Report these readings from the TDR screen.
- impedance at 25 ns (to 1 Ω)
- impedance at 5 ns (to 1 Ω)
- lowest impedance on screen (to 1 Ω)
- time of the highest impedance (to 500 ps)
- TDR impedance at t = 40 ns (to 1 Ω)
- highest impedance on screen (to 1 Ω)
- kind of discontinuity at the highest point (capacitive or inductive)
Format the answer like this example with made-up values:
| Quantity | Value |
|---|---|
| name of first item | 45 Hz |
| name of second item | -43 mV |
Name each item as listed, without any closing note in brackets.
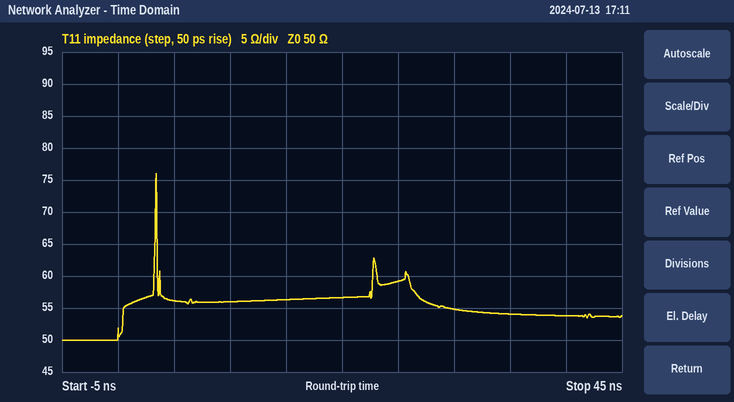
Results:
| Quantity | Value |
|---|---|
| impedance at 25 ns | 59 Ω |
| impedance at 5 ns | 56 Ω |
| lowest impedance on screen | 50 Ω |
| time of the highest impedance | 3.5 ns |
| TDR impedance at t = 40 ns | 54 Ω |
| highest impedance on screen | 76 Ω |
| kind of discontinuity at the highest point | inductive |
